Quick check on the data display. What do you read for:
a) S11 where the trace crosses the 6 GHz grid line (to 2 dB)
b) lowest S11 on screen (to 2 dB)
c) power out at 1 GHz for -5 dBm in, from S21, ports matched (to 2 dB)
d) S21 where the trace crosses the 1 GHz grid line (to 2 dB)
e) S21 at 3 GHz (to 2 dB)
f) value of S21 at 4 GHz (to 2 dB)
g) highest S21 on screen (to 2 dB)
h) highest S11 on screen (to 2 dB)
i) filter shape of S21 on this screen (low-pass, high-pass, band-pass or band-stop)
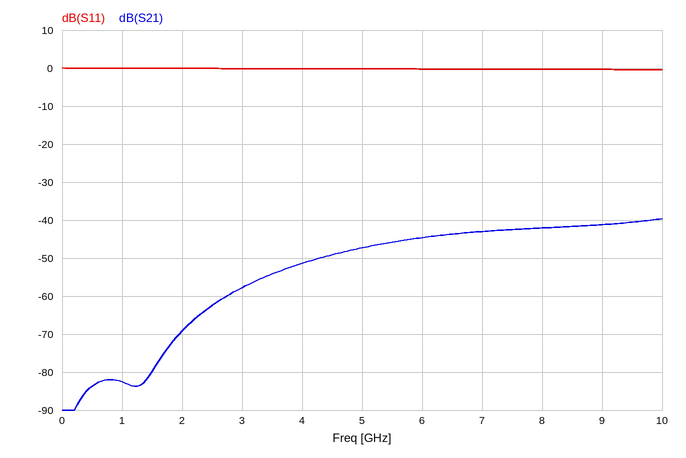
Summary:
0 dB
0 dB
-88 dBm
-82 dB
-58 dB
-52 dB
-40 dB
0 dB
high-pass
